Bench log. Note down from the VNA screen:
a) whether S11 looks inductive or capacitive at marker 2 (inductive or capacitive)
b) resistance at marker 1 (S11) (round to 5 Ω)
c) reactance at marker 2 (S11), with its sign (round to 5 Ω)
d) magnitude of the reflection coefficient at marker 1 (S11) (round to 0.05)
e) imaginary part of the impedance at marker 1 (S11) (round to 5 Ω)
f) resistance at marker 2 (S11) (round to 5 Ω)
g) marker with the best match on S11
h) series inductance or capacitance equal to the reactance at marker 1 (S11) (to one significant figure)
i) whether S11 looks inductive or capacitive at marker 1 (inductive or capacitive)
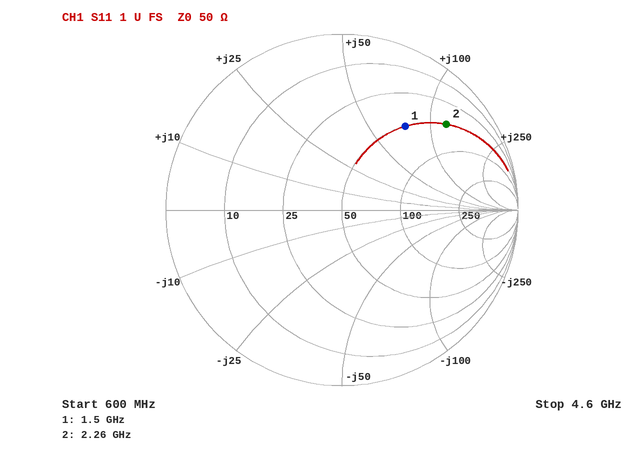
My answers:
inductive
50 Ω
+120 Ω
0.60
+75 Ω
50 Ω
marker 1
8 nH
inductive
